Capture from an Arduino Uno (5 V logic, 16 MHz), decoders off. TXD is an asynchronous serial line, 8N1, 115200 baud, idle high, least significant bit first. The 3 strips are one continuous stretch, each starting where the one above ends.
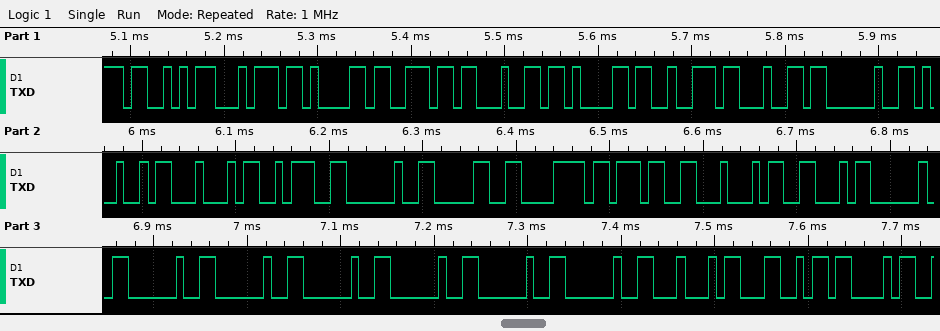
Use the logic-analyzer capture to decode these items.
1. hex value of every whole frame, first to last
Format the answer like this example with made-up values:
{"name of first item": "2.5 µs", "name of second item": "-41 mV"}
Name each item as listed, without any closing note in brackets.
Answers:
{"hex value of every whole frame, first to last": "53 74 61 6E 64 61 72 64 20 49 44 3A 20 30 78 37 44 46 20 20 20 20 20 20 20 44 4C 43"}
